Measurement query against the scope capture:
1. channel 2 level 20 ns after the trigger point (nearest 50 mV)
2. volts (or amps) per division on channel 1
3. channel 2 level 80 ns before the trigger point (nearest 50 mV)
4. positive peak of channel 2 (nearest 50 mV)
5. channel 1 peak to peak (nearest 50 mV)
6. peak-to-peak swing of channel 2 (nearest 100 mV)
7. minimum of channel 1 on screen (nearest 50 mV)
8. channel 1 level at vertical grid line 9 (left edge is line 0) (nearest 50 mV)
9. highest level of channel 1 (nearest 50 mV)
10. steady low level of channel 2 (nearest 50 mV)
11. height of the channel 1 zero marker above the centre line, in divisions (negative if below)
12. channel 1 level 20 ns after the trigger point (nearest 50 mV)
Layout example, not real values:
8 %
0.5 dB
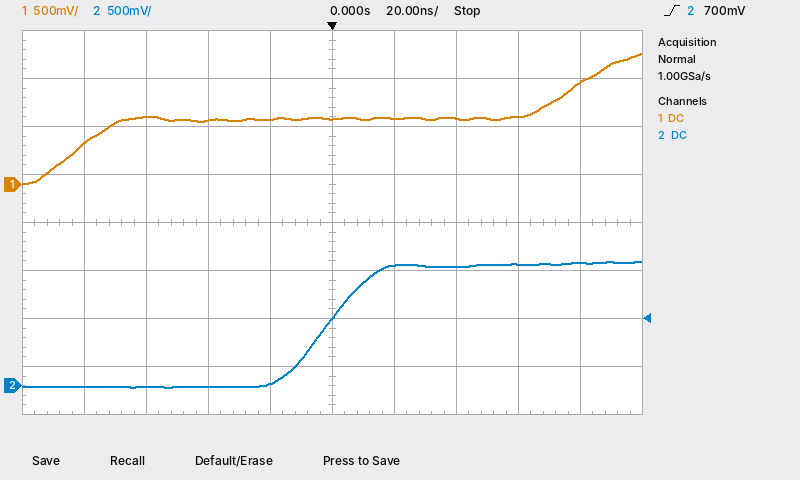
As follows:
1.25 V
500 mV
0 mV
1.30 V
1.35 V
1.30 V
0 mV
1.05 V
1.35 V
0 mV
+0.8 div
700 mV
